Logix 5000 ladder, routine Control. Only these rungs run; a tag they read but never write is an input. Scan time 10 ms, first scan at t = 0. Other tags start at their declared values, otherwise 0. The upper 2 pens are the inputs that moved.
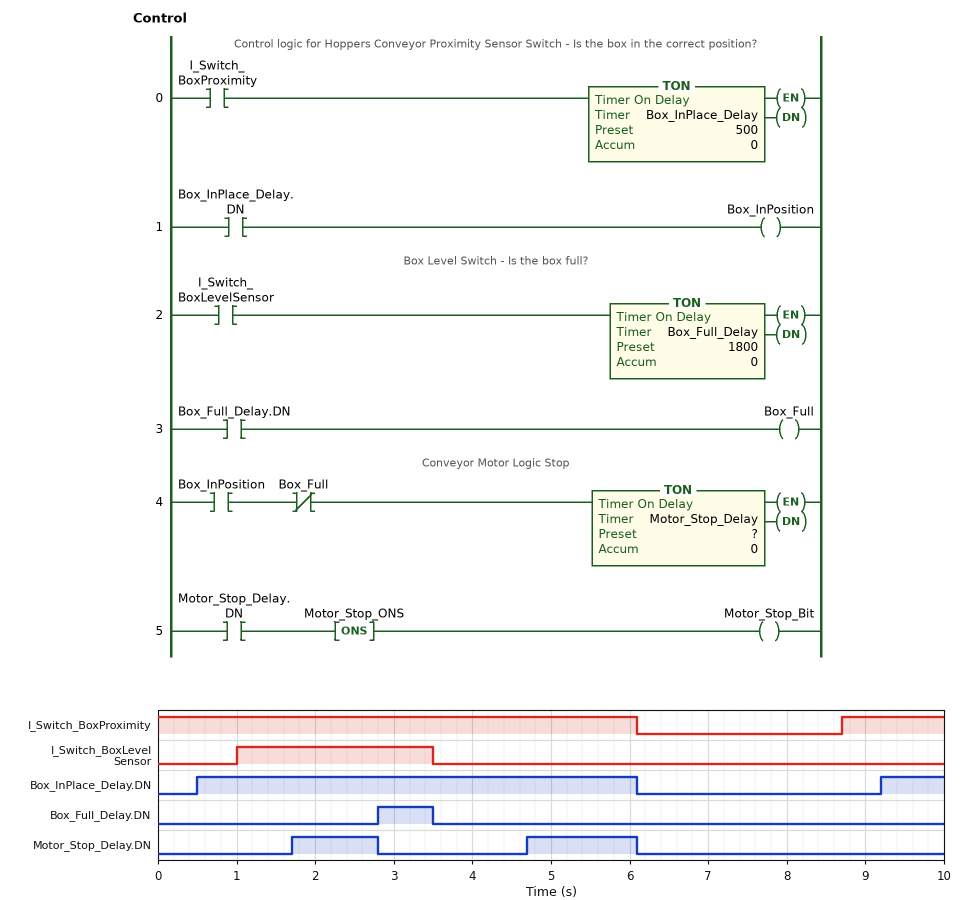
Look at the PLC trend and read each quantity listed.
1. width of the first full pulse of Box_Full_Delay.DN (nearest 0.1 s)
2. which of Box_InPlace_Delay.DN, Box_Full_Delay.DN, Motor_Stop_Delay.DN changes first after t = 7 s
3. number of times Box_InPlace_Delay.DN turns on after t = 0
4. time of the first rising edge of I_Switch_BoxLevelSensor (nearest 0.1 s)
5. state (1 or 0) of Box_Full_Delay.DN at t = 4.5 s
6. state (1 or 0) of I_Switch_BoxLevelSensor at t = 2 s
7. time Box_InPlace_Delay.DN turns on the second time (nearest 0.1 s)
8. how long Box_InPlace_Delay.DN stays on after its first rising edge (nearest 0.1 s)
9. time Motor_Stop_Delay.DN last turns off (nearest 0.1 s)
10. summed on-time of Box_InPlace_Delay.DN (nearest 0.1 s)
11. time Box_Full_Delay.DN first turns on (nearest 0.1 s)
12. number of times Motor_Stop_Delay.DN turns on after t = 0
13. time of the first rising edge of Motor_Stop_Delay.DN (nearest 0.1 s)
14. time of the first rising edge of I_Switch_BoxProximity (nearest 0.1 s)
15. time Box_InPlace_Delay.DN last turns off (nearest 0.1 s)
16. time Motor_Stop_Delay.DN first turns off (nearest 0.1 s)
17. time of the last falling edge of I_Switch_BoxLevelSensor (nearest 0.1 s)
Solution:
0.7 s
Box_InPlace_Delay.DN
2
1.0 s
0
1
9.2 s
5.6 s
6.1 s
6.4 s
2.8 s
2
1.7 s
8.7 s
6.1 s
2.8 s
3.5 s
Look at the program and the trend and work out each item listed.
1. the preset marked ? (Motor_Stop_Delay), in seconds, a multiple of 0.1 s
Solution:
1.2 s
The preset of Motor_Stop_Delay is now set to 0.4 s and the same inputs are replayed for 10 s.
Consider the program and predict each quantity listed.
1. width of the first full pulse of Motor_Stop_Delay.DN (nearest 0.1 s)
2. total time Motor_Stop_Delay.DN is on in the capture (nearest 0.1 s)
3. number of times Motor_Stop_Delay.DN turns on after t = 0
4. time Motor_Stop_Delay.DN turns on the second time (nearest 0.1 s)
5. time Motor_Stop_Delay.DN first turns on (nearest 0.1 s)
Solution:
1.9 s
4.5 s
3
3.9 s
0.9 s
